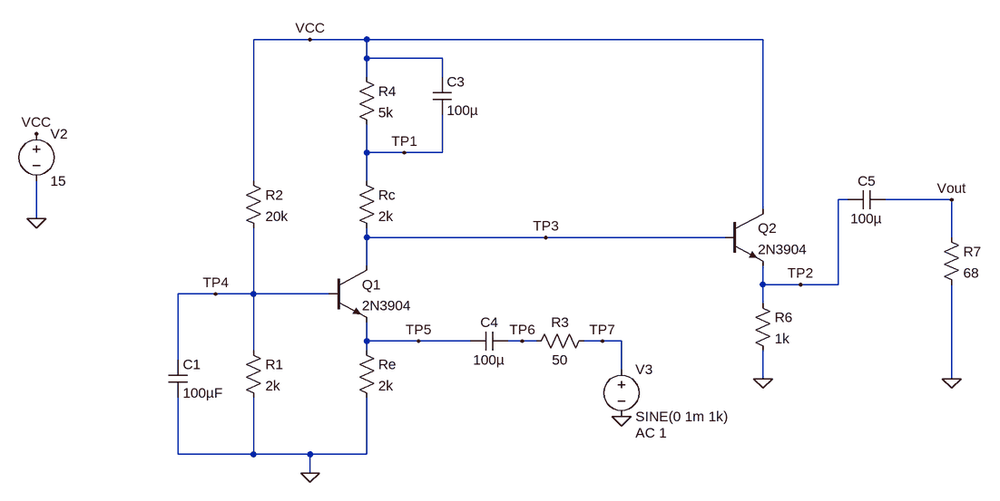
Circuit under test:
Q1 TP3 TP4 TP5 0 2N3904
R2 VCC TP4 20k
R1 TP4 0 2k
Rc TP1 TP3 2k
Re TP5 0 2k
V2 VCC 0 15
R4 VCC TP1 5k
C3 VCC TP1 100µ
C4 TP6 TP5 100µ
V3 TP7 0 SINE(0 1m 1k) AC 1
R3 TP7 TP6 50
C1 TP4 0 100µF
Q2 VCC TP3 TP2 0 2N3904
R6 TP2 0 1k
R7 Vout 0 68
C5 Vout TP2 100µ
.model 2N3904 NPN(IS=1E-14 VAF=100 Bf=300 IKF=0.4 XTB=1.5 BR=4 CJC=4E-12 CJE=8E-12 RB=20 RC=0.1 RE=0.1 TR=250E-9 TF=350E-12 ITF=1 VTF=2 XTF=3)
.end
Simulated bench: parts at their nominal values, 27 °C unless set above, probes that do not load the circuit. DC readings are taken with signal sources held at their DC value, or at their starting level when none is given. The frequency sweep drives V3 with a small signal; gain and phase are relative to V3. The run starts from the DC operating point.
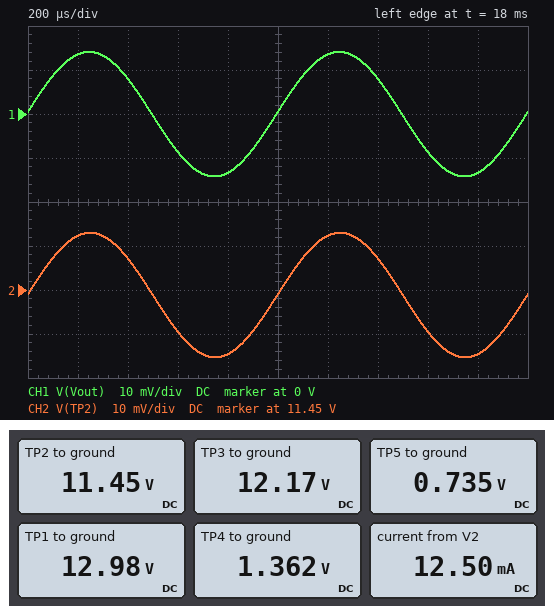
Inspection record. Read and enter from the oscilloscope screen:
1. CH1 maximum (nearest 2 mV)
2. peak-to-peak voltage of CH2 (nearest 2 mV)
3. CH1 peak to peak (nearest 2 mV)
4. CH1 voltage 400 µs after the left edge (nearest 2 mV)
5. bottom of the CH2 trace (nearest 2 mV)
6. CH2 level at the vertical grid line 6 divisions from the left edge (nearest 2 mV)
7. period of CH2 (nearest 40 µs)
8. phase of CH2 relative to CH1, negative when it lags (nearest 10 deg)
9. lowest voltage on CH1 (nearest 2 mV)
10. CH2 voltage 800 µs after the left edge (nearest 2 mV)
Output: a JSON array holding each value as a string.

["14 mV", "28 mV", "28 mV", "8 mV", "11.434 V", "11.462 V", "1.00 ms", "0 deg", "-14 mV", "11.436 V"]
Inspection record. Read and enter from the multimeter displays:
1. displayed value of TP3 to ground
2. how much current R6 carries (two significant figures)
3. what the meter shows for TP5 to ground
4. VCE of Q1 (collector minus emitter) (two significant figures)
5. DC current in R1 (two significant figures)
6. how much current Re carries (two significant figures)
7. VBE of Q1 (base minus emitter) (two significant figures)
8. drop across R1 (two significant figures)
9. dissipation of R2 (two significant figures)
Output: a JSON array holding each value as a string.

["12.17 V", "11 mA", "0.735 V", "11 V", "680 µA", "370 µA", "630 mV", "1.4 V", "9.3 mW"]
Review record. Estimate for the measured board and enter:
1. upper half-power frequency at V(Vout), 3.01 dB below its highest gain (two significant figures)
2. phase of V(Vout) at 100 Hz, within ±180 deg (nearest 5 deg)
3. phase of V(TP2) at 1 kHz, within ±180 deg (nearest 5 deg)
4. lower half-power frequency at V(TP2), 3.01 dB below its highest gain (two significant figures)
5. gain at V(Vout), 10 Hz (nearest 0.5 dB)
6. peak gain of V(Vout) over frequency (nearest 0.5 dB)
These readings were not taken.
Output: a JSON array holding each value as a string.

["8.6 MHz", "20 deg", "0 deg", "11 Hz", "11.5 dB", "23.0 dB"]
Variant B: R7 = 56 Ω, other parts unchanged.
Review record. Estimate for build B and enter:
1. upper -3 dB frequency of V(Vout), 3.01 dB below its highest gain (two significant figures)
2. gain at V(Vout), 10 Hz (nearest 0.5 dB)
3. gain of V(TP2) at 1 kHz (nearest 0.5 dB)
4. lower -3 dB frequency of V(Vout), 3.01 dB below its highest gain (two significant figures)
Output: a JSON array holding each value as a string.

["7.9 MHz", "10.0 dB", "23.0 dB", "30 Hz"]
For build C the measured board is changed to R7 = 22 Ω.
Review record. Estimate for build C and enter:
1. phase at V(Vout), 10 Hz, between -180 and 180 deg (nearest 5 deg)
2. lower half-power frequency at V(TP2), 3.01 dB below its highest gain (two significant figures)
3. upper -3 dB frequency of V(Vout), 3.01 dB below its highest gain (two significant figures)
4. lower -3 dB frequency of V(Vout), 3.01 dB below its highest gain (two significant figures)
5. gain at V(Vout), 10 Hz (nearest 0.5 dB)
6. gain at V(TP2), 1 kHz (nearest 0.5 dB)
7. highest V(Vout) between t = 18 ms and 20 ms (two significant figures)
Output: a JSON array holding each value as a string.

["130 deg", "10 Hz", "5.0 MHz", "54 Hz", "2.5 dB", "21.0 dB", "11 mV"]
